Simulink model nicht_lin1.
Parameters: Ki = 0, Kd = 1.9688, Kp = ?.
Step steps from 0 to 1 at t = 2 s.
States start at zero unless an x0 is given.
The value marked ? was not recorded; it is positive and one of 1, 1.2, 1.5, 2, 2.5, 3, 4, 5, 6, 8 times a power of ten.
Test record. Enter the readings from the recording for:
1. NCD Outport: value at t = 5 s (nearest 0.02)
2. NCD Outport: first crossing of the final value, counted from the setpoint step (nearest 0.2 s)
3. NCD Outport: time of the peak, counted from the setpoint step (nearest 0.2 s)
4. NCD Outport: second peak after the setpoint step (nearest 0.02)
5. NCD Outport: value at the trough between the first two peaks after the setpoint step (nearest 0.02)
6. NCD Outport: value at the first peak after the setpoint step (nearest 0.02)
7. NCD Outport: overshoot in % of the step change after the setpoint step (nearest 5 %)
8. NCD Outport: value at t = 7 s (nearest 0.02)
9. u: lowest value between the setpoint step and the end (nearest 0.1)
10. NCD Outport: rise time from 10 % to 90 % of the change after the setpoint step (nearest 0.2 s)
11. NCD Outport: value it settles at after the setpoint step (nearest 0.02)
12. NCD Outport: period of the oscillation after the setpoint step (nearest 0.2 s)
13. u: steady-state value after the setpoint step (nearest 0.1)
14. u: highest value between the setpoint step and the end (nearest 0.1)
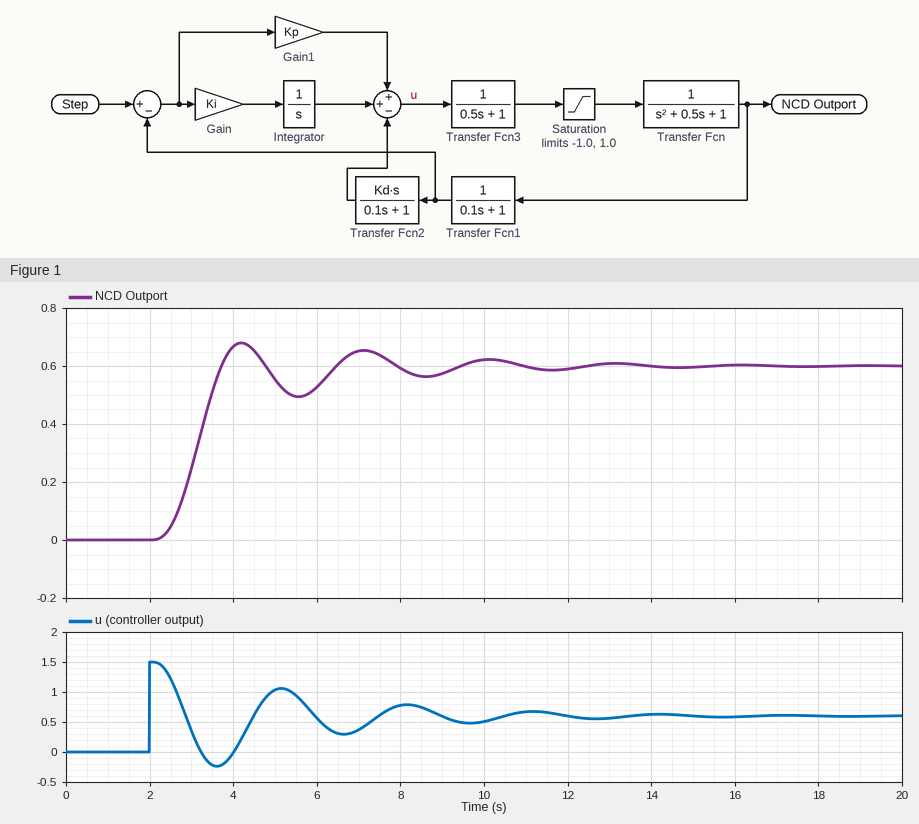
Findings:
0.56
1.8 s
2.2 s
0.66
0.50
0.68
15 %
0.66
-0.2
1.0 s
0.60
3.0 s
0.6
1.5
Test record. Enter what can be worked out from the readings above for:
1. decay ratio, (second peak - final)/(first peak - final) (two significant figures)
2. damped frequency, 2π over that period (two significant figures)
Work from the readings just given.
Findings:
0.75
2.1 rad/s
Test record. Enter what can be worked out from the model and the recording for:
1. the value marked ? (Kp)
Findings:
1.5
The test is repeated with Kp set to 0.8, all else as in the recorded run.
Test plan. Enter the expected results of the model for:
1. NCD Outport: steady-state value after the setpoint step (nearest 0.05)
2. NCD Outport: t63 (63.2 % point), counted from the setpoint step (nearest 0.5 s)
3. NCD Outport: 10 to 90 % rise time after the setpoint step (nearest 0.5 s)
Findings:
0.45
1.5 s
1.5 s
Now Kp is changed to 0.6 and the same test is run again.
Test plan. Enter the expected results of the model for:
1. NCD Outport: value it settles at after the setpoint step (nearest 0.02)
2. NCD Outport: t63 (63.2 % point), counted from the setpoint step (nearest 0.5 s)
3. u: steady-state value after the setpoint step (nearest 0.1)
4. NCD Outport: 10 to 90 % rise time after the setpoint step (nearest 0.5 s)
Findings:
0.38
1.5 s
0.4
3.5 s
